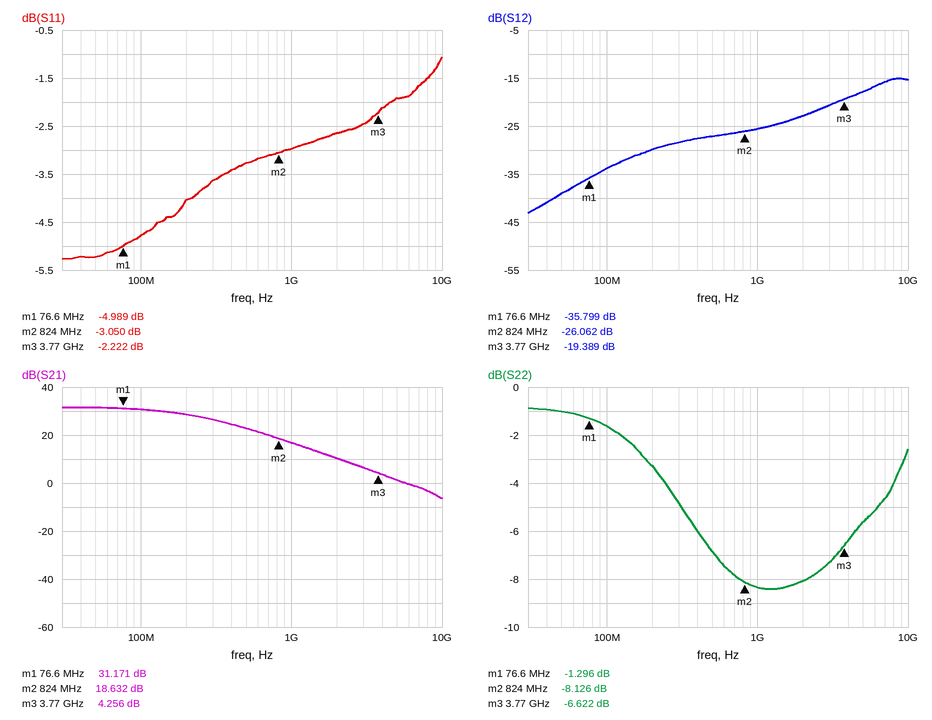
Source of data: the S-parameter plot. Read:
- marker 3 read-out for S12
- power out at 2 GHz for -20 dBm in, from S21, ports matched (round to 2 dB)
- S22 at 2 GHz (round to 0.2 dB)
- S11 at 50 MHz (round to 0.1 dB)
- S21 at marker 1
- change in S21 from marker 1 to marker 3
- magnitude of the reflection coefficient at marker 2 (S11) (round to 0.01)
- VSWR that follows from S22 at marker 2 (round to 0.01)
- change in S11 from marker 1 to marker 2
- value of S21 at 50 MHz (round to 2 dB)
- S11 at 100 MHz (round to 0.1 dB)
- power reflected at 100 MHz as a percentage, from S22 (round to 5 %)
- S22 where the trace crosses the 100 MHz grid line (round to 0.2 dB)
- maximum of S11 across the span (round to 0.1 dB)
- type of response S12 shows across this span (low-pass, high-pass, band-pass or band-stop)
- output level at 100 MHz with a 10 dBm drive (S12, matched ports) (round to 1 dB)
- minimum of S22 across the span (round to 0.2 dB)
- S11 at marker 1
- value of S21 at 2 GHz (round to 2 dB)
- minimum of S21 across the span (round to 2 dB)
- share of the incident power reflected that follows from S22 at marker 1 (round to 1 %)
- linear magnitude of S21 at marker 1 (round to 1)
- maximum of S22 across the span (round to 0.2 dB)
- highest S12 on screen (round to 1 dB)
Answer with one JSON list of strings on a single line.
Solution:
["-19.389 dB", "-10 dBm", "-8.0 dB", "-5.2 dB", "31.171 dB", "-26.915 dB", "0.70", "2.29", "1.939 dB", "32 dB", "-4.8 dB", "70 %", "-1.6 dB", "-1.1 dB", "high-pass", "-24 dBm", "-8.4 dB", "-4.989 dB", "10 dB", "-6 dB", "74 %", "36", "-0.8 dB", "-15 dB"]
